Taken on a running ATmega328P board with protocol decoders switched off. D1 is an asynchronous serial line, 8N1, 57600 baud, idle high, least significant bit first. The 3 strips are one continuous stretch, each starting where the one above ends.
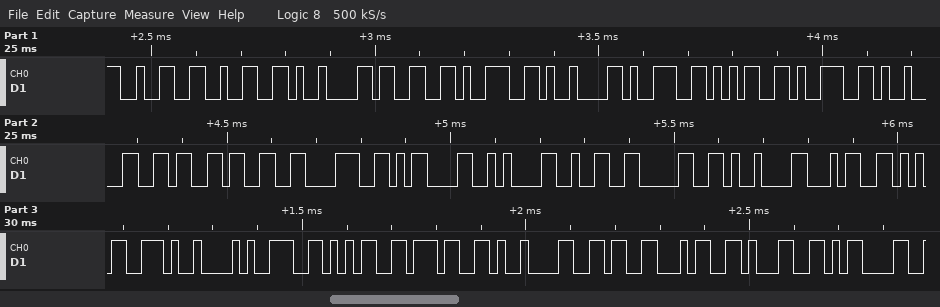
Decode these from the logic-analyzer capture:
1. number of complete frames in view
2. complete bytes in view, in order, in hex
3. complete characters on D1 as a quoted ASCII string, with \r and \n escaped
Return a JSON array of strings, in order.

["29", "32 32 09 33 39 09 39 35 39 09 36 33 38 0D 0A 32 30 09 34 35 09 39 35 37 09 36 34 31 0D", "\"22\\t39\\t959\\t638\\r\\n20\\t45\\t957\\t641\\r\""]
